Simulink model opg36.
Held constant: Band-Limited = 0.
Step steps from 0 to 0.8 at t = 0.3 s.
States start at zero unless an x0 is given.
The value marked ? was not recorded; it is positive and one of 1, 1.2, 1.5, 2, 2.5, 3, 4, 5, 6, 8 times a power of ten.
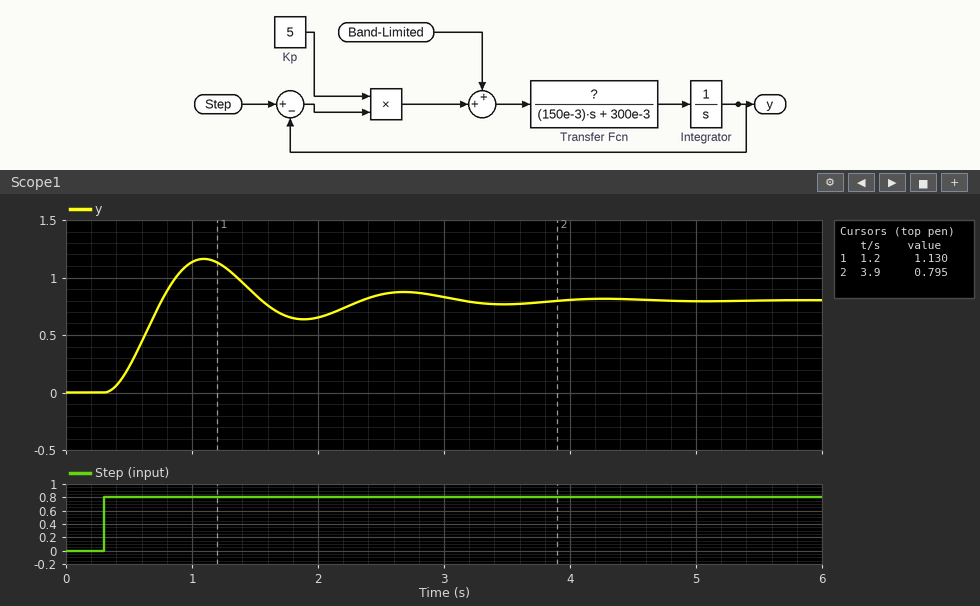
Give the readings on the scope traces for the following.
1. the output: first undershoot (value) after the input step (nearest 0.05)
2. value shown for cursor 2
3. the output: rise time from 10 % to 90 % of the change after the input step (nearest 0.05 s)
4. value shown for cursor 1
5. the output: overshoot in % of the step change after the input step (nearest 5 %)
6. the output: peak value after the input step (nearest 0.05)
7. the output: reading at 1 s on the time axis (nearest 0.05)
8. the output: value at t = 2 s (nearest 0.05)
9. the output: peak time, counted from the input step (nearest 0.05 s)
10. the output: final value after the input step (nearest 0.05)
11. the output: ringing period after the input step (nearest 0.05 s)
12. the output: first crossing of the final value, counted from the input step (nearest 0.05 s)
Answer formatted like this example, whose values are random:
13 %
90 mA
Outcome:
0.65
0.795
0.30 s
1.130
45 %
1.15
1.15
0.65
0.80 s
0.80
1.60 s
0.45 s
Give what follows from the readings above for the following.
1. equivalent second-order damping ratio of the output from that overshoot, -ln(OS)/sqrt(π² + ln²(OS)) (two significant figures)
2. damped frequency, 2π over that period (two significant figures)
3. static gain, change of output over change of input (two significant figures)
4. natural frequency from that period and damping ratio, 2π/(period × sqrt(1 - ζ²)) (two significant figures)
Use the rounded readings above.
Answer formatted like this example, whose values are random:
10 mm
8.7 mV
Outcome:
0.25
3.9 rad/s
1.0
4.1 rad/s
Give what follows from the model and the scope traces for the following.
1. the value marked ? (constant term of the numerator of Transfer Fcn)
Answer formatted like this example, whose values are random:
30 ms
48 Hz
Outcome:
0.5
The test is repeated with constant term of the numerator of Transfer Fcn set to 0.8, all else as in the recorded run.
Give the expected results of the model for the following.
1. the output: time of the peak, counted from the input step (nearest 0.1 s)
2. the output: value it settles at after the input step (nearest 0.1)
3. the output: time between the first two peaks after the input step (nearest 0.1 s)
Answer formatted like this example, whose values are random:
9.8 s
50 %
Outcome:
0.6 s
0.8
1.2 s
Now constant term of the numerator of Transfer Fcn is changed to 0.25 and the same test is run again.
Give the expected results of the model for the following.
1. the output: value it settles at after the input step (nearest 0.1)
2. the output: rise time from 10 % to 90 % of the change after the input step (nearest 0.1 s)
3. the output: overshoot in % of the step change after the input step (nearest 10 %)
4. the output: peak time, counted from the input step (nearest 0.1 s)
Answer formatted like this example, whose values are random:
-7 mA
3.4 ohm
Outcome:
0.8
0.5 s
30 %
1.2 s
